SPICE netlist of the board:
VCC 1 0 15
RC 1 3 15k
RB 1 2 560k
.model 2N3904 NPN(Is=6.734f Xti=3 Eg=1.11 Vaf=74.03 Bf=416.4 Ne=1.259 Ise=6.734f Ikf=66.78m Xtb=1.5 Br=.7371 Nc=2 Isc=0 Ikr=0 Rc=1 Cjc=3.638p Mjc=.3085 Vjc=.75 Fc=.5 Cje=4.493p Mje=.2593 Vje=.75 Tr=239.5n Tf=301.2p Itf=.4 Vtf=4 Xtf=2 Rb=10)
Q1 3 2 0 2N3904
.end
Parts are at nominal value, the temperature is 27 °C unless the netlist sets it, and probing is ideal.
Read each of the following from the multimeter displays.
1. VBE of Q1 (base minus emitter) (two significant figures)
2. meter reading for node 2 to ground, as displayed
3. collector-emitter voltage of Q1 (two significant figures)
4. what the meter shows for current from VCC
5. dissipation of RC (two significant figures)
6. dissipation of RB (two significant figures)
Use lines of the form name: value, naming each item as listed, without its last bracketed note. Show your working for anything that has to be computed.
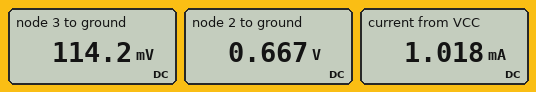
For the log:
VBE of Q1 (base minus emitter): 667 mV = 670 mV
meter reading for node 2 to ground, as displayed: 0.667 V
collector-emitter voltage of Q1: 114.2 mV = 110 mV
what the meter shows for current from VCC: 1.018 mA
dissipation of RC: (15 V - 114.2 mV)^2 / 15 kΩ = 15 mW
dissipation of RB: (15 V - 667 mV)^2 / 560 kΩ = 370 µW
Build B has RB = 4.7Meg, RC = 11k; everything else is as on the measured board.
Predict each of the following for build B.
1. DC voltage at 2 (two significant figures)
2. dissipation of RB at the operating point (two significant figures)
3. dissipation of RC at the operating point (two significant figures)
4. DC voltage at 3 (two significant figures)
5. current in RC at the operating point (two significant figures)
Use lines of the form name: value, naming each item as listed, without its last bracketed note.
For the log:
DC voltage at 2: 640 mV
dissipation of RB at the operating point: 44 µW
dissipation of RC at the operating point: 1.8 mW
DC voltage at 3: 11 V
current in RC at the operating point: 400 µA
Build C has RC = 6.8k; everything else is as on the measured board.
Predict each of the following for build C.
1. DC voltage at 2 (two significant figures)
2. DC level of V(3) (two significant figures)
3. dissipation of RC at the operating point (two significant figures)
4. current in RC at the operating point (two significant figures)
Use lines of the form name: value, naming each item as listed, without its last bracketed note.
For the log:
DC voltage at 2: 690 mV
DC level of V(3): 150 mV
dissipation of RC at the operating point: 32 mW
current in RC at the operating point: 2.2 mA
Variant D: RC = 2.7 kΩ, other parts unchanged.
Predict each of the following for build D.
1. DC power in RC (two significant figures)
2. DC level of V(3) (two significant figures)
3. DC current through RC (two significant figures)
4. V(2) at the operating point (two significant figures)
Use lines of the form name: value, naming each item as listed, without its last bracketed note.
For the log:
DC power in RC: 45 mW
DC level of V(3): 4.0 V
DC current through RC: 4.1 mA
V(2) at the operating point: 700 mV
